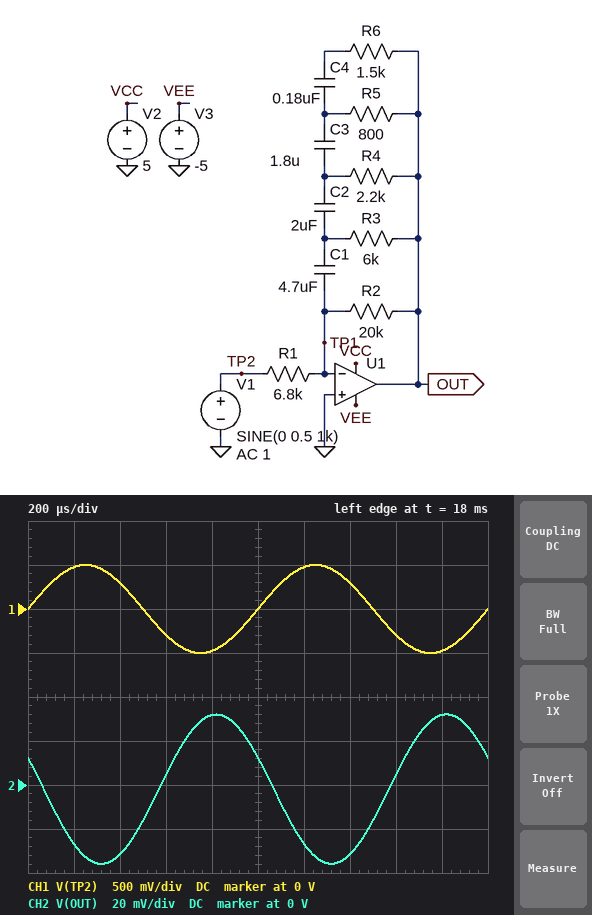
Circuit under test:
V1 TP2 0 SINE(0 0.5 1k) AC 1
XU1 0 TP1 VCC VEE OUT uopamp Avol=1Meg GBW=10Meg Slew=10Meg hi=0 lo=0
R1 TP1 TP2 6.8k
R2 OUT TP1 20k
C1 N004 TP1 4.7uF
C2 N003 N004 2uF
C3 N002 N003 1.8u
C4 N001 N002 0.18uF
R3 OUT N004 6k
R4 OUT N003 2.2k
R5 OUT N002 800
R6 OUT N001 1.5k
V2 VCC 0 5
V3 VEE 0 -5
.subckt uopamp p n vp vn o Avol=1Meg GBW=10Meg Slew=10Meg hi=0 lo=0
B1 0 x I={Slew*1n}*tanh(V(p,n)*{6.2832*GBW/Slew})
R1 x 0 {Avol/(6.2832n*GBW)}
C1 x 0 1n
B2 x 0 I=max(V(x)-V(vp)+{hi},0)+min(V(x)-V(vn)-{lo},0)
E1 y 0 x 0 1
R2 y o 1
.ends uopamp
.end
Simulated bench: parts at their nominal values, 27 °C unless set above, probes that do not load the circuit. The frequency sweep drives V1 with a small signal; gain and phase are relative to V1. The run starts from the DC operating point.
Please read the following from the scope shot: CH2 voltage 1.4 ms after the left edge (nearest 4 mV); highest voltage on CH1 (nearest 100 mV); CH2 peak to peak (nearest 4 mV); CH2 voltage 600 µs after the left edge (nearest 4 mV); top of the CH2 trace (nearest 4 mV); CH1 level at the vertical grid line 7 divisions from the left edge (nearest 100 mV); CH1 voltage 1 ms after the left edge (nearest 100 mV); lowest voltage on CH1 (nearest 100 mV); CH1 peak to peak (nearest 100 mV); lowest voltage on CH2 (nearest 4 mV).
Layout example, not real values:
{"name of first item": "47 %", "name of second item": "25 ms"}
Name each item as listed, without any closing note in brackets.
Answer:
{"CH2 voltage 1.4 ms after the left edge": "-32 mV", "highest voltage on CH1": "500 mV", "CH2 peak to peak": "68 mV", "CH2 voltage 600 µs after the left edge": "4 mV", "top of the CH2 trace": "32 mV", "CH1 level at the vertical grid line 7 divisions from the left edge": "300 mV", "CH1 voltage 1 ms after the left edge": "0 V", "lowest voltage on CH1": "-500 mV", "CH1 peak to peak": "1.0 V", "lowest voltage on CH2": "-36 mV"}
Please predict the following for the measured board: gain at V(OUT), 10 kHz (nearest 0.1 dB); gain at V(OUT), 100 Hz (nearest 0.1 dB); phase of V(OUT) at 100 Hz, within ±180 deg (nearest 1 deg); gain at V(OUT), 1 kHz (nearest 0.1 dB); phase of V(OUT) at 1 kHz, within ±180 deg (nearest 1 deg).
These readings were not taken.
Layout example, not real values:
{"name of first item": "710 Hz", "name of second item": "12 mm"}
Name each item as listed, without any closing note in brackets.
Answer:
{"gain at V(OUT), 10 kHz": "-24.9 dB", "gain at V(OUT), 100 Hz": "-13.2 dB", "phase of V(OUT) at 100 Hz, within ±180 deg": "126 deg", "gain at V(OUT), 1 kHz": "-23.4 dB", "phase of V(OUT) at 1 kHz, within ±180 deg": "155 deg"}
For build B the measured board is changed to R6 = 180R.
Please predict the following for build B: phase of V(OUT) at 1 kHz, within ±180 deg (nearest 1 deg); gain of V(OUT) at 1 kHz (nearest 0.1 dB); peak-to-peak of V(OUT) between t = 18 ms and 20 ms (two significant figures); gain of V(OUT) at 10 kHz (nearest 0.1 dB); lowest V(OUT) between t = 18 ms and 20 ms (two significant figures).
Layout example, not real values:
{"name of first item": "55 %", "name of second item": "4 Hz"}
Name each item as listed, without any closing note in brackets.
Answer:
{"phase of V(OUT) at 1 kHz, within ±180 deg": "140 deg", "gain of V(OUT) at 1 kHz": "-22.3 dB", "peak-to-peak of V(OUT) between t = 18 ms and 20 ms": "77 mV", "gain of V(OUT) at 10 kHz": "-32.8 dB", "lowest V(OUT) between t = 18 ms and 20 ms": "-40 mV"}
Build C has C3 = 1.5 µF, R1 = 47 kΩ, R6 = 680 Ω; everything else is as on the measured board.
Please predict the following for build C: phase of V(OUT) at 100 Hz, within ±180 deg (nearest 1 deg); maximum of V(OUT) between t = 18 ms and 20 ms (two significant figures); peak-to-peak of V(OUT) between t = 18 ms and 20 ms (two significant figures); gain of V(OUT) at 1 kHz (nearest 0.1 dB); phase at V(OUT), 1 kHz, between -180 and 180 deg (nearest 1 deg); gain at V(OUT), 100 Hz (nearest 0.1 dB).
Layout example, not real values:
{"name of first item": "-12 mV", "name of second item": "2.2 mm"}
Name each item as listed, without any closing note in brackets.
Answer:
{"phase of V(OUT) at 100 Hz, within ±180 deg": "127 deg", "maximum of V(OUT) between t = 18 ms and 20 ms": "4.8 mV", "peak-to-peak of V(OUT) between t = 18 ms and 20 ms": "10 mV", "gain of V(OUT) at 1 kHz": "-39.9 dB", "phase at V(OUT), 1 kHz, between -180 and 180 deg": "146 deg", "gain at V(OUT), 100 Hz": "-29.7 dB"}
